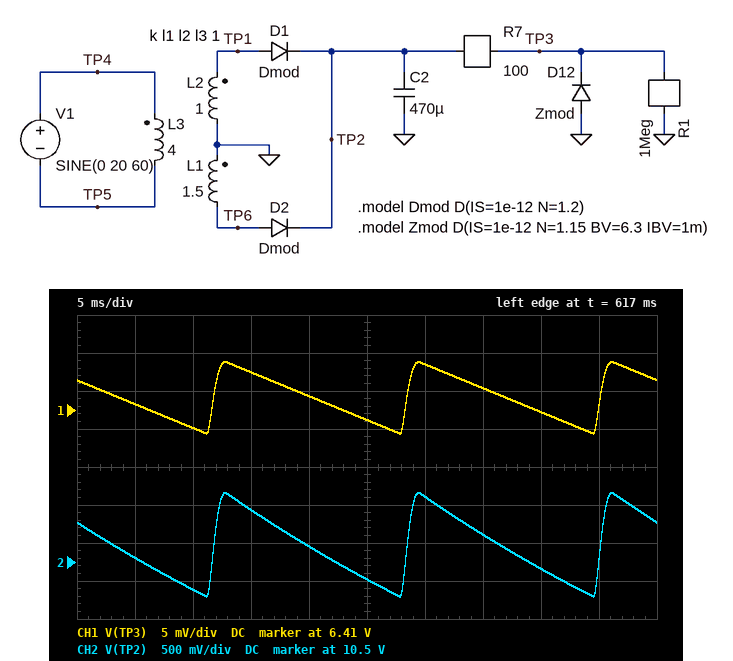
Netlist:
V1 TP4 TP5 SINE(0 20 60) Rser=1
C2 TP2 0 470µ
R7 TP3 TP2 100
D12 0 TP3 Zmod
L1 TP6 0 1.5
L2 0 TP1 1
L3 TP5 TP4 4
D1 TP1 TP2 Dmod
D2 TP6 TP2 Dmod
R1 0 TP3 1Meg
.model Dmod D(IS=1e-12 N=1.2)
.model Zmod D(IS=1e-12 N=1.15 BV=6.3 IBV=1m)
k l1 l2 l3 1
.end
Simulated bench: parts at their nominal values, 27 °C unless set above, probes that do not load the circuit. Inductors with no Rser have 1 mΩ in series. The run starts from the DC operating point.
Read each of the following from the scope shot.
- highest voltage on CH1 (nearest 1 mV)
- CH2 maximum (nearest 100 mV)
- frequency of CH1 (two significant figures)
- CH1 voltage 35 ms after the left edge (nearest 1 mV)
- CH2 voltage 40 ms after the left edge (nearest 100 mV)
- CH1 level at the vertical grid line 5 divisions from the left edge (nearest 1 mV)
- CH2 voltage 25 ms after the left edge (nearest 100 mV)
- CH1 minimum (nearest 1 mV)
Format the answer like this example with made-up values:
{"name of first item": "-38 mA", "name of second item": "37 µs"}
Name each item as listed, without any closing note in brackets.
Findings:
{"highest voltage on CH1": "6.416 V", "CH2 maximum": "11.4 V", "frequency of CH1": "60 Hz", "CH1 voltage 35 ms after the left edge": "6.413 V", "CH2 voltage 40 ms after the left edge": "10.4 V", "CH1 level at the vertical grid line 5 divisions from the left edge": "6.409 V", "CH2 voltage 25 ms after the left edge": "10.3 V", "CH1 minimum": "6.407 V"}
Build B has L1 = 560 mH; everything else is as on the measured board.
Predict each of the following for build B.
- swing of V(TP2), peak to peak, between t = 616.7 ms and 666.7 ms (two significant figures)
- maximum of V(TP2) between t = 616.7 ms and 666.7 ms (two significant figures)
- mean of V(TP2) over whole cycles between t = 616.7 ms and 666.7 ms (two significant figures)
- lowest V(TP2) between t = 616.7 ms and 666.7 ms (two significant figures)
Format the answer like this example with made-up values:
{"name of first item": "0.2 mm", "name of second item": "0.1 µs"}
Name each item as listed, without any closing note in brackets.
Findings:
{"swing of V(TP2), peak to peak, between t = 616.7 ms and 666.7 ms": "770 mV", "maximum of V(TP2) between t = 616.7 ms and 666.7 ms": "9.2 V", "mean of V(TP2) over whole cycles between t = 616.7 ms and 666.7 ms": "8.8 V", "lowest V(TP2) between t = 616.7 ms and 666.7 ms": "8.4 V"}
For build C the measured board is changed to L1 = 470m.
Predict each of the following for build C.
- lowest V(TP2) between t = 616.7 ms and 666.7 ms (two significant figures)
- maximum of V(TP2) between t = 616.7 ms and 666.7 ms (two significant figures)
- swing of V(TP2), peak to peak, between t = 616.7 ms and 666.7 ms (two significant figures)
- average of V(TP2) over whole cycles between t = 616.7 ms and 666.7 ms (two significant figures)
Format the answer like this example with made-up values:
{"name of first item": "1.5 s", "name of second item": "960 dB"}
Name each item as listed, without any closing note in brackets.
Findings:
{"lowest V(TP2) between t = 616.7 ms and 666.7 ms": "8.4 V", "maximum of V(TP2) between t = 616.7 ms and 666.7 ms": "9.2 V", "swing of V(TP2), peak to peak, between t = 616.7 ms and 666.7 ms": "770 mV", "average of V(TP2) over whole cycles between t = 616.7 ms and 666.7 ms": "8.8 V"}
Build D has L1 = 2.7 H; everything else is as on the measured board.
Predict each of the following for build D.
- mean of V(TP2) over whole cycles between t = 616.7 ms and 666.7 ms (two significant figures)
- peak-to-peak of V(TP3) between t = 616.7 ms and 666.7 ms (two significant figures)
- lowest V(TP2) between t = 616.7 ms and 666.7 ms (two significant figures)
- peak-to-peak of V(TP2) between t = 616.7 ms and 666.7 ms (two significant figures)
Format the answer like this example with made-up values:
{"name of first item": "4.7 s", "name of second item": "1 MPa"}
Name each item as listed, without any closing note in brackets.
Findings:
{"mean of V(TP2) over whole cycles between t = 616.7 ms and 666.7 ms": "14 V", "peak-to-peak of V(TP3) between t = 616.7 ms and 666.7 ms": "9.3 mV", "lowest V(TP2) between t = 616.7 ms and 666.7 ms": "13 V", "peak-to-peak of V(TP2) between t = 616.7 ms and 666.7 ms": "2.4 V"}
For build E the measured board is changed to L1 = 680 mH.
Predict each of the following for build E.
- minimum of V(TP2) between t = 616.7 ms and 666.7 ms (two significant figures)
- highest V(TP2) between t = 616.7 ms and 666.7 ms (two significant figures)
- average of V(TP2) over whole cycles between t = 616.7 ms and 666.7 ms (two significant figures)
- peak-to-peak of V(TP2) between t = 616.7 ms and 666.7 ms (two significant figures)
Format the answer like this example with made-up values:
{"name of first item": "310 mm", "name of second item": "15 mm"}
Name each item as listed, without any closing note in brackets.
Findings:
{"minimum of V(TP2) between t = 616.7 ms and 666.7 ms": "8.4 V", "highest V(TP2) between t = 616.7 ms and 666.7 ms": "9.2 V", "average of V(TP2) over whole cycles between t = 616.7 ms and 666.7 ms": "8.8 V", "peak-to-peak of V(TP2) between t = 616.7 ms and 666.7 ms": "770 mV"}
